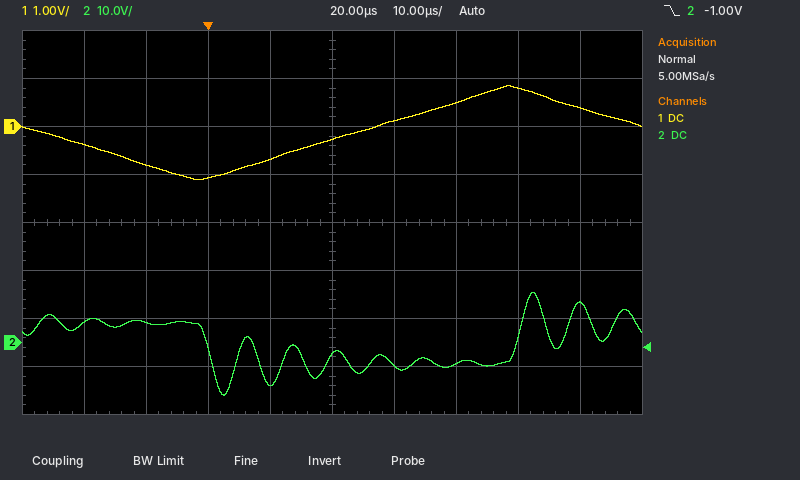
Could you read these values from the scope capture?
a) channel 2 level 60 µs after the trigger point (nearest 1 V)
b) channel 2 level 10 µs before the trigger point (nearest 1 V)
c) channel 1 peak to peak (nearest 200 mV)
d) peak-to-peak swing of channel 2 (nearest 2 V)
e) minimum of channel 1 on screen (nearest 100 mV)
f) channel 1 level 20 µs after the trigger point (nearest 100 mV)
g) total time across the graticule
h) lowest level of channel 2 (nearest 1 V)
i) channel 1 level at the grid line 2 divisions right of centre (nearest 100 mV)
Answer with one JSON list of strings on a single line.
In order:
["8 V", "4 V", "2.0 V", "22 V", "-1.1 V", "-300 mV", "100 µs", "-11 V", "500 mV"]
